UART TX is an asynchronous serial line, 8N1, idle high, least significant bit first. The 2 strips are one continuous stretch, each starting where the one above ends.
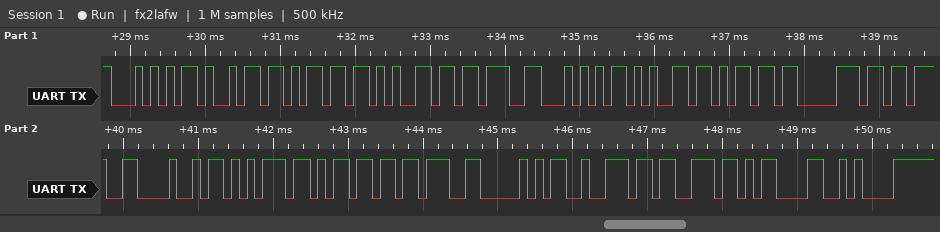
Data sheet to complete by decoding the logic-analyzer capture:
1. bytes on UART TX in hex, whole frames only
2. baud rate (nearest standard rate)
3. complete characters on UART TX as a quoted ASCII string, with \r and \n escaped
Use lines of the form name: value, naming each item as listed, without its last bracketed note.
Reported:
bytes on UART TX in hex, whole frames only: 0x54 0x69 0x6D 0x65 0x3B 0x54 0x65 0x6D 0x70 0x3B 0x48 0x75 0x6D 0x3B 0x50 0x72 0x73 0x0D 0x0A
baud rate: 9600 baud
complete characters on UART TX as a quoted ASCII string, with \r and \n escaped: "Time;Temp;Hum;Prs\r\n"
